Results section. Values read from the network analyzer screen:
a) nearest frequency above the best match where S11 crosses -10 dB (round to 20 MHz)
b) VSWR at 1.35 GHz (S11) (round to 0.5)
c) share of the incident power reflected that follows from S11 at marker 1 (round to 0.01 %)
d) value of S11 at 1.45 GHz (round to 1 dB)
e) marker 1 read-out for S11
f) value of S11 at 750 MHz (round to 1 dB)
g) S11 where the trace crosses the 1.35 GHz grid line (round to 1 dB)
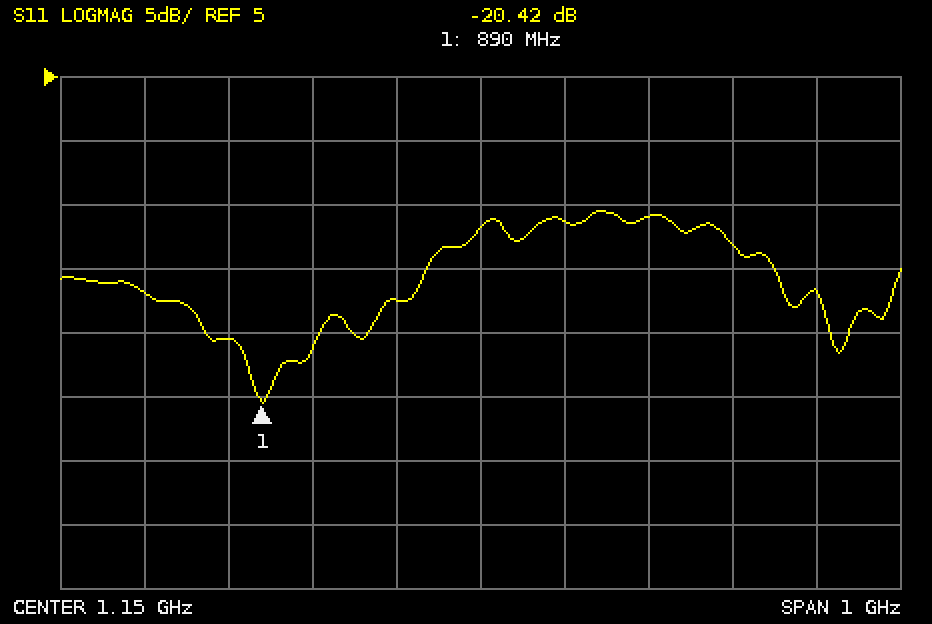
1.08 GHz
3.0
0.91 %
-8 dB
-20.42 dB
-12 dB
-6 dB
